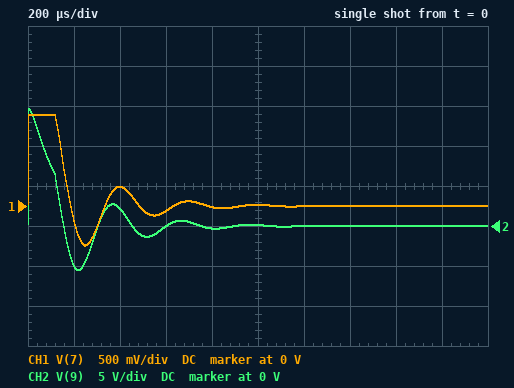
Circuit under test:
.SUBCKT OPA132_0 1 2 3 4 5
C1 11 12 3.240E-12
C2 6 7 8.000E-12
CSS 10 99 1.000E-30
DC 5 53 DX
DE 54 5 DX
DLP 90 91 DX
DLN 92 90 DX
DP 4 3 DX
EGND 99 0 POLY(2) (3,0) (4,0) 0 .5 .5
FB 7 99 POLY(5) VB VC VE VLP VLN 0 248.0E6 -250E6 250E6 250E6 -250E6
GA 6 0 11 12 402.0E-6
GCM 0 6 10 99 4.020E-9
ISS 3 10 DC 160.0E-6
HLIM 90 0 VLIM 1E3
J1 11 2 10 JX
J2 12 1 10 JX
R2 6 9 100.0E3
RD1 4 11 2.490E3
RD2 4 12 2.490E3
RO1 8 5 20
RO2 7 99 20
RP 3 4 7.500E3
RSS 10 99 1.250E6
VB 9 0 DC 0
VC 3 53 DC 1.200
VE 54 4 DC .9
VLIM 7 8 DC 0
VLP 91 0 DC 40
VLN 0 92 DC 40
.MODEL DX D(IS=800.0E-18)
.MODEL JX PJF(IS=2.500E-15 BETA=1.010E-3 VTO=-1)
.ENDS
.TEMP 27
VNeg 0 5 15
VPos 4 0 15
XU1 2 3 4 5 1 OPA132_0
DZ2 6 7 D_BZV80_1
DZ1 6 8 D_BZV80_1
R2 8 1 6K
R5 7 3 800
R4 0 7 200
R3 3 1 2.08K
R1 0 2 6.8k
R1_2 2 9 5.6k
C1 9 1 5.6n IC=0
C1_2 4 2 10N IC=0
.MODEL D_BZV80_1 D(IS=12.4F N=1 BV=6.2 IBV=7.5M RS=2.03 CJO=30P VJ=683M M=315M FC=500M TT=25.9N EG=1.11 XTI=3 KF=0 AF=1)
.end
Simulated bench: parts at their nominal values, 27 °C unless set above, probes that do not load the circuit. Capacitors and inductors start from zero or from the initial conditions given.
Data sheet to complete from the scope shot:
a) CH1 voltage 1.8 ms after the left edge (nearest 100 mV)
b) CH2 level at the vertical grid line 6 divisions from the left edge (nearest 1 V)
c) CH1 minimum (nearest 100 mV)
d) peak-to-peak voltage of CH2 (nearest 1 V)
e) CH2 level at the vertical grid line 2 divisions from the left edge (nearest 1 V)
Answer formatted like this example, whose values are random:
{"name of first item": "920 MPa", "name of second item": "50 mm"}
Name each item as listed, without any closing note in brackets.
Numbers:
{"CH1 voltage 1.8 ms after the left edge": "0 V", "CH2 level at the vertical grid line 6 divisions from the left edge": "0 V", "CH1 minimum": "-500 mV", "peak-to-peak voltage of CH2": "20 V", "CH2 level at the vertical grid line 2 divisions from the left edge": "2 V"}
